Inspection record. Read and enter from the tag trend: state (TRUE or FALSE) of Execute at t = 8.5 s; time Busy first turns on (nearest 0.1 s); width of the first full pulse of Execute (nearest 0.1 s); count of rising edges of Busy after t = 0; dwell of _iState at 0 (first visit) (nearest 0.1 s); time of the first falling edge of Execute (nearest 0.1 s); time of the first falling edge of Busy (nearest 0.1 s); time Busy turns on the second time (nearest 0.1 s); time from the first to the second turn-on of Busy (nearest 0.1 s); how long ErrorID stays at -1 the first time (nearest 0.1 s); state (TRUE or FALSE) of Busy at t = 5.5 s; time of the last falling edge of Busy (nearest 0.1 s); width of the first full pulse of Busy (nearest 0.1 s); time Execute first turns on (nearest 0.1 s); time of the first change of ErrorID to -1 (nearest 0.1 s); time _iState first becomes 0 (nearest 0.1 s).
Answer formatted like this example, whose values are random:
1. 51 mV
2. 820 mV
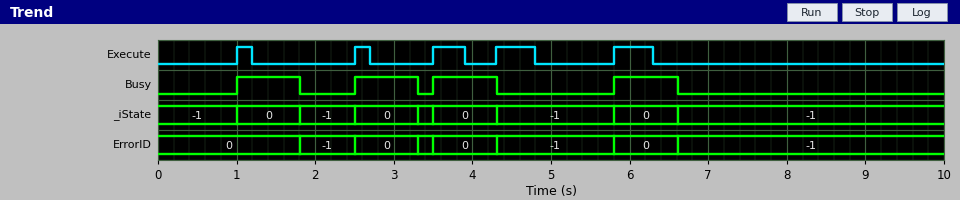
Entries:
1. FALSE
2. 1.0 s
3. 0.2 s
4. 4
5. 0.8 s
6. 1.2 s
7. 1.8 s
8. 2.5 s
9. 1.5 s
10. 0.7 s
11. FALSE
12. 6.6 s
13. 0.8 s
14. 1.0 s
15. 1.8 s
16. 1.0 s
